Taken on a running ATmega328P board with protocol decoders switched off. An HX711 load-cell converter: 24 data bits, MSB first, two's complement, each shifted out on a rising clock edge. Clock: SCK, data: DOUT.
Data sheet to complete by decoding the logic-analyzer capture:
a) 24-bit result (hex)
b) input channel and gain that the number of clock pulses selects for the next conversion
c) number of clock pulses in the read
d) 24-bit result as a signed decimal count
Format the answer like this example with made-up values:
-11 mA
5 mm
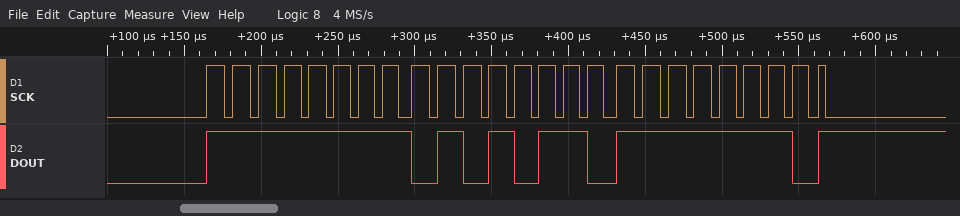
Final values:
0xFF56FE
channel A, gain 128
25
-43266
